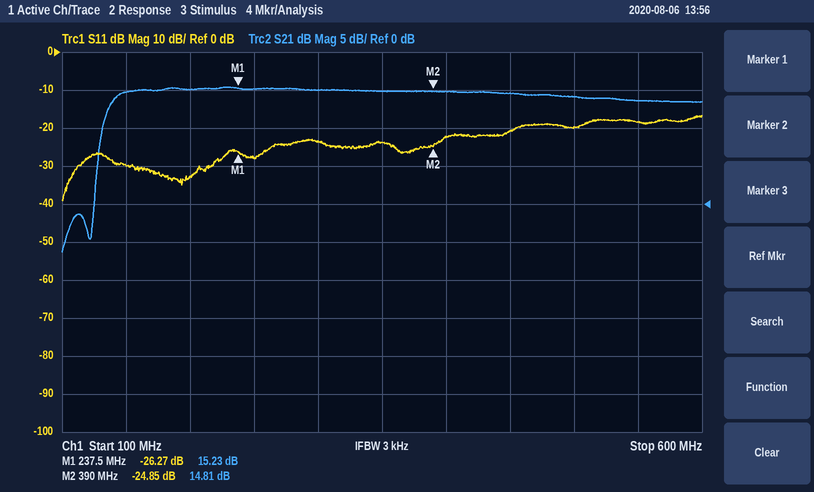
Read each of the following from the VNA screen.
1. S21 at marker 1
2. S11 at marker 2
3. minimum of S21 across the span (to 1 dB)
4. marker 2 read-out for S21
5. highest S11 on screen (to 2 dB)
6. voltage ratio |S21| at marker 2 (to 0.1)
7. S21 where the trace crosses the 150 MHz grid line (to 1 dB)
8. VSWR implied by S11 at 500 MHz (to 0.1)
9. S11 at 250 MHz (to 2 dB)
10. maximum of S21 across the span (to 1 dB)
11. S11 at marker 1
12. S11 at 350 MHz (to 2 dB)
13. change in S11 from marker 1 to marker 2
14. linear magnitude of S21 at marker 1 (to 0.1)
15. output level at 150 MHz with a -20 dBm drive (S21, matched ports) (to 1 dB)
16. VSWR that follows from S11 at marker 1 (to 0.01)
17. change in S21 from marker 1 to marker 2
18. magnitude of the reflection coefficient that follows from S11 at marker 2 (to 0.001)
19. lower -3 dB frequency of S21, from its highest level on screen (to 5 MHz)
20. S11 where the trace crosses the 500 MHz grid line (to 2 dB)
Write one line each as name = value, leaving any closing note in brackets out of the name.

S21 at marker 1 = 15.23 dB
S11 at marker 2 = -24.85 dB
minimum of S21 across the span = -6 dB
marker 2 read-out for S21 = 14.81 dB
highest S11 on screen = -16 dB
voltage ratio |S21| at marker 2 = 5.5
S21 where the trace crosses the 150 MHz grid line = 15 dB
VSWR implied by S11 at 500 MHz = 1.2
S11 at 250 MHz = -28 dB
maximum of S21 across the span = 15 dB
S11 at marker 1 = -26.27 dB
S11 at 350 MHz = -24 dB
change in S11 from marker 1 to marker 2 = 1.42 dB
linear magnitude of S21 at marker 1 = 5.8
output level at 150 MHz with a -20 dBm drive (S21, matched ports) = -5 dBm
VSWR that follows from S11 at marker 1 = 1.10
change in S21 from marker 1 to marker 2 = -0.42 dB
magnitude of the reflection coefficient that follows from S11 at marker 2 = 0.057
lower -3 dB frequency of S21, from its highest level on screen = 135 MHz
S11 where the trace crosses the 500 MHz grid line = -20 dB
